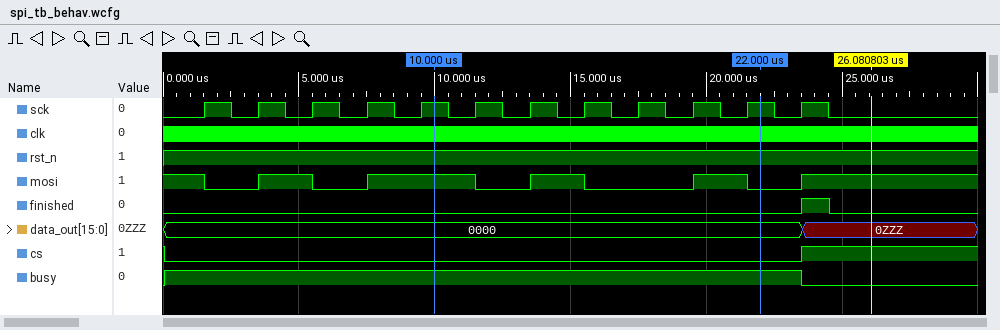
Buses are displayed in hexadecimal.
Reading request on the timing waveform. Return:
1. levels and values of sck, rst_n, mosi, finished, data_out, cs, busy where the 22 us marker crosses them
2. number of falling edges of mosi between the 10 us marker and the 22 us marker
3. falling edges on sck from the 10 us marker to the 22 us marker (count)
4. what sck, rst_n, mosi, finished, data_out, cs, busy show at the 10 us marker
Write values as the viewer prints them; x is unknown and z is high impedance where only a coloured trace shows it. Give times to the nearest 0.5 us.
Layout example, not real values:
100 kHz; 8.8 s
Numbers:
sck=1, rst_n=1, mosi=0, finished=0, data_out=0000, cs=0, busy=1; 3; 6; sck=1, rst_n=1, mosi=1, finished=0, data_out=0000, cs=0, busy=1
